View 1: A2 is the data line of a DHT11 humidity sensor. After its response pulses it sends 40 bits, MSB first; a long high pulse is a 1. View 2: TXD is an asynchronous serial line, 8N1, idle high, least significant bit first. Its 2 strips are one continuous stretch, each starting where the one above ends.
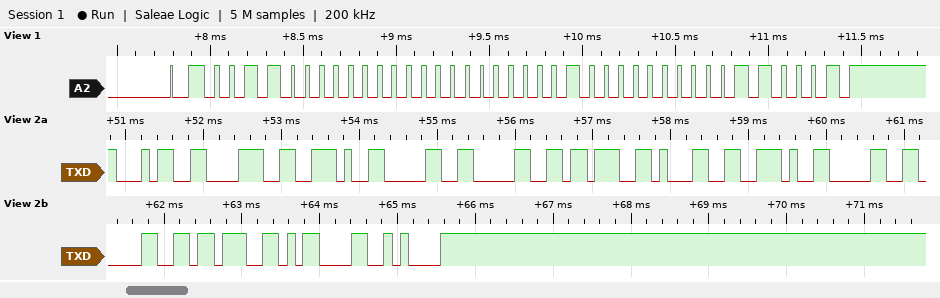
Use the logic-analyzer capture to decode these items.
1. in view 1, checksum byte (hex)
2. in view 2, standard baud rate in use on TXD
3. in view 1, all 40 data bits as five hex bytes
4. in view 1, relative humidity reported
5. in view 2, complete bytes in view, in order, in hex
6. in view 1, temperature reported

0x31
9600 baud
30 00 01 00 31
48 %
0x34 0x38 0x2E 0x30 0x30 0x3B 0x31 0x2E 0x30 0x30 0x3B 0x0D 0x0A
1.0 °C
